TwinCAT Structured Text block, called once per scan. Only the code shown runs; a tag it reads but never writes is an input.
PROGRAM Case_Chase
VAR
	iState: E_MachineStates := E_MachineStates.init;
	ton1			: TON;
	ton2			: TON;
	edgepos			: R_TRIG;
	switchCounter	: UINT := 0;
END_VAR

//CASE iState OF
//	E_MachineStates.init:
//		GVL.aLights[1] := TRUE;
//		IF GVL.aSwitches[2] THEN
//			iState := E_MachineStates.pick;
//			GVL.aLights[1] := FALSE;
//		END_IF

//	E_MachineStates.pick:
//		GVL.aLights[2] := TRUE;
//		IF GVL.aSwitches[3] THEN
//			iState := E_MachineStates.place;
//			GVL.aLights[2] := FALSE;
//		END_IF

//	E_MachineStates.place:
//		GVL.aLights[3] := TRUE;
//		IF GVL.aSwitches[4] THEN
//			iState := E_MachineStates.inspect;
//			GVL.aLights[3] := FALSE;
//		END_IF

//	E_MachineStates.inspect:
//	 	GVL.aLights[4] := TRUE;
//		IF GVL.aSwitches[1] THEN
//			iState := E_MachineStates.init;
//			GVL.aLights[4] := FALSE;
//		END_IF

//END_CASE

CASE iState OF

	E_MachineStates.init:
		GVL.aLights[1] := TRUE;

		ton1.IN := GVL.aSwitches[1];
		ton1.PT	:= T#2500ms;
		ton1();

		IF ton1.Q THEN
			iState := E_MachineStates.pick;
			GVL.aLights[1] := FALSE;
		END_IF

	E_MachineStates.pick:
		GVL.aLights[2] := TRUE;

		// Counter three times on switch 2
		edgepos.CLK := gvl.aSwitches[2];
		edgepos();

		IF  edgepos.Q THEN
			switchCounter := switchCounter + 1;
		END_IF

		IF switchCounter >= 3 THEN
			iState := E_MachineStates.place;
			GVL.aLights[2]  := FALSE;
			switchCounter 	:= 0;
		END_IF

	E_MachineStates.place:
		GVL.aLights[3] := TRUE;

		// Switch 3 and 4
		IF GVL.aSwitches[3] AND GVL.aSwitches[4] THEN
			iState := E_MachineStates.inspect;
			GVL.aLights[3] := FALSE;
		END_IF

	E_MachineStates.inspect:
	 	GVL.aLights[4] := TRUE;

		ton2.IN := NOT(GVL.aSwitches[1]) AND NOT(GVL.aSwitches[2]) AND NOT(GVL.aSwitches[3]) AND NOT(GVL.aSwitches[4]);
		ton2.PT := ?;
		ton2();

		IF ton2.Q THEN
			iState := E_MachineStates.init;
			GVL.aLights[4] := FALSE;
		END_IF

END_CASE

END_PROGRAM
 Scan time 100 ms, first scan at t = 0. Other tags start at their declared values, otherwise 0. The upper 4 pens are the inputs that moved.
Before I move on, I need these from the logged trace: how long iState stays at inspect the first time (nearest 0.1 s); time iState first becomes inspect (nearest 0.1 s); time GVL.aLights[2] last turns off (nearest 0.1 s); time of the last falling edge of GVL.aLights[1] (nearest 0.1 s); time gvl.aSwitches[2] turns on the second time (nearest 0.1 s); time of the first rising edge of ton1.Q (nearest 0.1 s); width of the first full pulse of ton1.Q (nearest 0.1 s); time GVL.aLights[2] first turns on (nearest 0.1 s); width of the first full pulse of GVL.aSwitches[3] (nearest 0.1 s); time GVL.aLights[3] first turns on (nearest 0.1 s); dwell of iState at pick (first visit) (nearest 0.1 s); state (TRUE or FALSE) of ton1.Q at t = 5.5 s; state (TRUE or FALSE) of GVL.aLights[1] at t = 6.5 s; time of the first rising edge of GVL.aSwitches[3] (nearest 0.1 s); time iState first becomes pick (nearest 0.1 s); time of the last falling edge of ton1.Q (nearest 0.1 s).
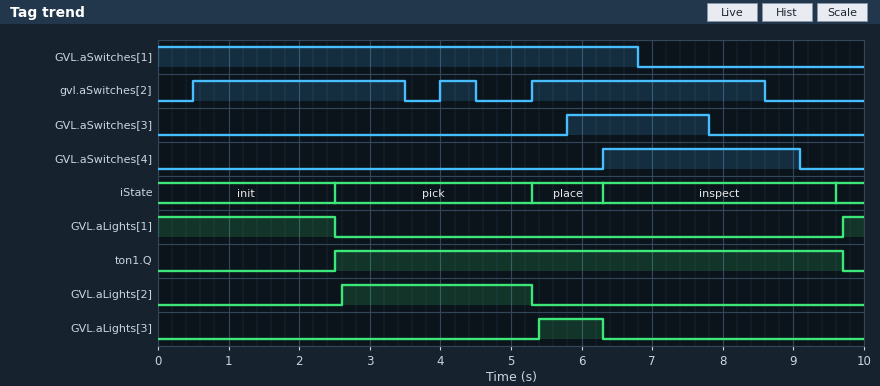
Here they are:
3.3 s
6.3 s
5.3 s
2.5 s
4.0 s
2.5 s
7.2 s
2.6 s
2.0 s
5.4 s
2.8 s
TRUE
FALSE
5.8 s
2.5 s
9.7 s
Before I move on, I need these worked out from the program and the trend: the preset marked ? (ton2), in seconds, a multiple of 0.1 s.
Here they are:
0.5 s
